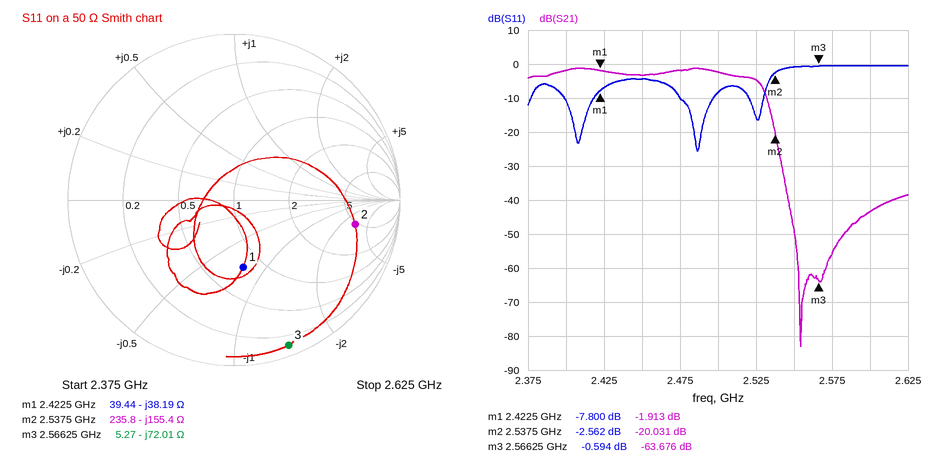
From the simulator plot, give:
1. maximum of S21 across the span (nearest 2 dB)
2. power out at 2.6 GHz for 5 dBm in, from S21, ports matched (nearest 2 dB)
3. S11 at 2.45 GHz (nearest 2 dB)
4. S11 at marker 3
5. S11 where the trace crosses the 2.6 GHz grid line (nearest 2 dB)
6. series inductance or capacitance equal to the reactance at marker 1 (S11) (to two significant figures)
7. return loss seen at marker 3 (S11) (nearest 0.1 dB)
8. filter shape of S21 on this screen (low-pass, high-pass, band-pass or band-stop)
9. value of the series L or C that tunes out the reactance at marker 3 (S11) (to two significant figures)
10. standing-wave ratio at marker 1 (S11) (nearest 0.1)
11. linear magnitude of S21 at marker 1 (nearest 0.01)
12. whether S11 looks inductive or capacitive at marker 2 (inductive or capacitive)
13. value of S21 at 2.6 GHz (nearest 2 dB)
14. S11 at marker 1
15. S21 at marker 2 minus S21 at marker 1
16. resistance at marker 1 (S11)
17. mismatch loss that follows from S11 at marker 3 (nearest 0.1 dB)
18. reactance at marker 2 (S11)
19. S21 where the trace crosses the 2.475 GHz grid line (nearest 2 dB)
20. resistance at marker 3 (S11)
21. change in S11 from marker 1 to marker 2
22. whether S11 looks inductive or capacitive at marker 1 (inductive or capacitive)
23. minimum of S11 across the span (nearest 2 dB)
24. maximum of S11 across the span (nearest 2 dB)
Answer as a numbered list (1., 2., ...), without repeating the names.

1. -2 dB
2. -38 dBm
3. -4 dB
4. -0.594 dB
5. 0 dB
6. 1.7 pF
7. 0.6 dB
8. low-pass
9. 4.5 nH
10. 2.4
11. 0.80
12. capacitive
13. -44 dB
14. -7.800 dB
15. -18.118 dB
16. 39.44 Ω
17. 8.9 dB
18. -155.4 Ω
19. -2 dB
20. 5.27 Ω
21. 5.238 dB
22. capacitive
23. -26 dB
24. 0 dB
